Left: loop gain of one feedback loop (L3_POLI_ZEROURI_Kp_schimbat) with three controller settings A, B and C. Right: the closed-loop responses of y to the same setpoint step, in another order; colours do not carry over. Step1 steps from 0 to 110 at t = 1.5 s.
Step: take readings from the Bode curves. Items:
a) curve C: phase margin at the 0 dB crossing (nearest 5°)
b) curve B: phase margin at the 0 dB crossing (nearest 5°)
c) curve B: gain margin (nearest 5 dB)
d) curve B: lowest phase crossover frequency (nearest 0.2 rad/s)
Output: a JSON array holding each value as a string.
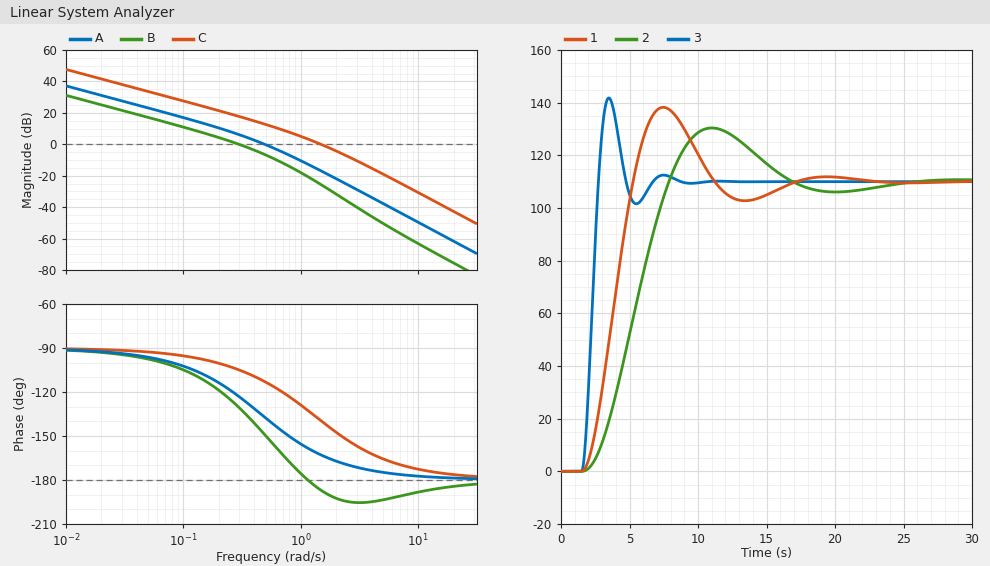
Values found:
["40°", "50°", "20 dB", "1.2 rad/s"]
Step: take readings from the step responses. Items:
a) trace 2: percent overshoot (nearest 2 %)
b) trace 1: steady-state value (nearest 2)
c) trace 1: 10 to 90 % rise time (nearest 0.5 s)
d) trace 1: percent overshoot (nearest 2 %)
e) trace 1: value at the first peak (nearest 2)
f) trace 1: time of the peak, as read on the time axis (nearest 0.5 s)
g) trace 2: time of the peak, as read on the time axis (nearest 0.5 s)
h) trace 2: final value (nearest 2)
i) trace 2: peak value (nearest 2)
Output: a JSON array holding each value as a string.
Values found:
["18 %", "110", "2.5 s", "26 %", "138", "7.5 s", "11.0 s", "110", "130"]
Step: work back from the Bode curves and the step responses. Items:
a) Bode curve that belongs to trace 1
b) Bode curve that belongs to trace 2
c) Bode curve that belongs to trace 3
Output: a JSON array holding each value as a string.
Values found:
["A", "B", "C"]
